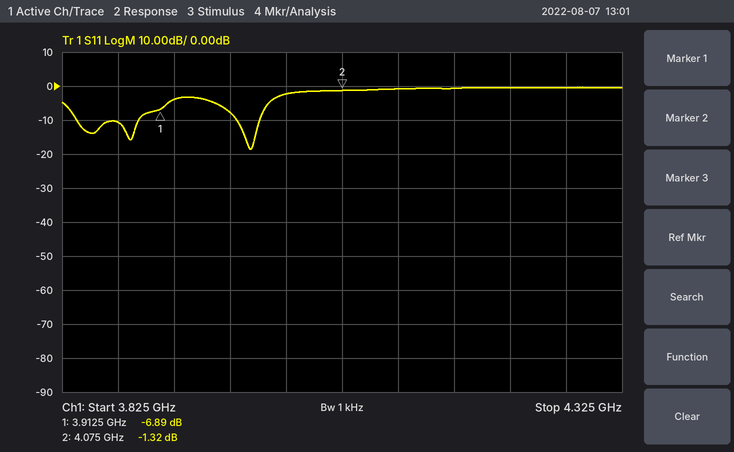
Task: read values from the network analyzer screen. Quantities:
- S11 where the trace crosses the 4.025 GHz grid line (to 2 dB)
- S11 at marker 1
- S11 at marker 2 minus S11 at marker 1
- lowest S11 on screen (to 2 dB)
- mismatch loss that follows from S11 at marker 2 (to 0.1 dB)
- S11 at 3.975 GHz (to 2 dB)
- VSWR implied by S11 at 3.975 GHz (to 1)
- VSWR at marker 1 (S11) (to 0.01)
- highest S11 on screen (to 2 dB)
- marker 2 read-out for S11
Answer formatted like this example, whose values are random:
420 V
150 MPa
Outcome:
-2 dB
-6.89 dB
5.57 dB
-18 dB
5.8 dB
-8 dB
2
2.65
0 dB
-1.32 dB
